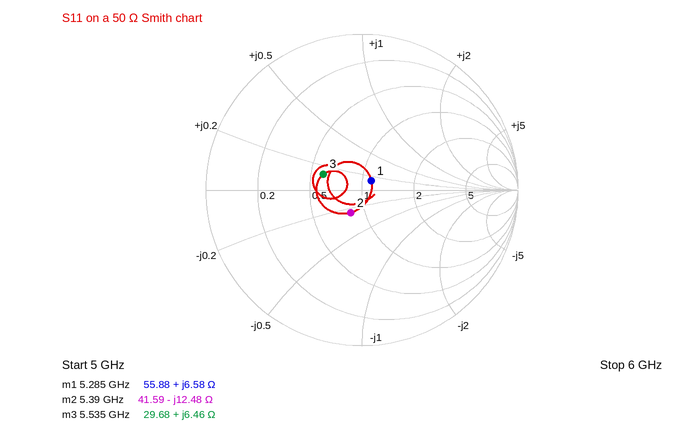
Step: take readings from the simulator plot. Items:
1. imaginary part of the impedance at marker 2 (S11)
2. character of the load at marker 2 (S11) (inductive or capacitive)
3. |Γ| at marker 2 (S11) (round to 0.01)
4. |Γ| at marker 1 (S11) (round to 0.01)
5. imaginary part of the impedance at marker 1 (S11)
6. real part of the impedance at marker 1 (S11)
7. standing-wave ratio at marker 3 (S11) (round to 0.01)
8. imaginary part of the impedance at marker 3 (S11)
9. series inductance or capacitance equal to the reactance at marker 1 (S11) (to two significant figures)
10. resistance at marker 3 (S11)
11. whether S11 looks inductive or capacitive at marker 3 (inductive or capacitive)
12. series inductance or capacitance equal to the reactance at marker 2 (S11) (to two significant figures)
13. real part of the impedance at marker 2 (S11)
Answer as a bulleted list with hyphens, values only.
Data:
- -12.48 Ω
- capacitive
- 0.16
- 0.08
- +6.58 Ω
- 55.88 Ω
- 1.73
- +6.46 Ω
- 200 pH
- 29.68 Ω
- inductive
- 2.4 pF
- 41.59 Ω
